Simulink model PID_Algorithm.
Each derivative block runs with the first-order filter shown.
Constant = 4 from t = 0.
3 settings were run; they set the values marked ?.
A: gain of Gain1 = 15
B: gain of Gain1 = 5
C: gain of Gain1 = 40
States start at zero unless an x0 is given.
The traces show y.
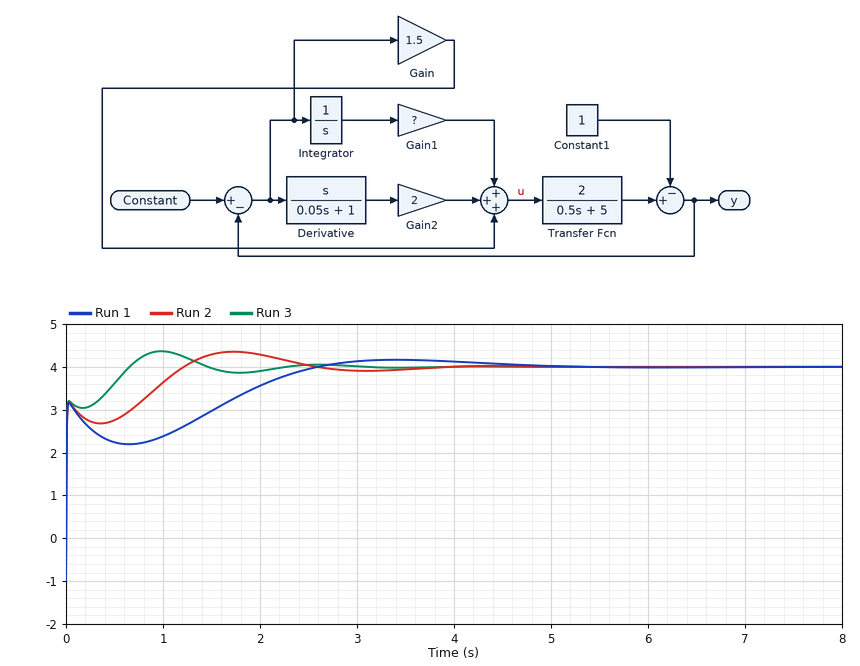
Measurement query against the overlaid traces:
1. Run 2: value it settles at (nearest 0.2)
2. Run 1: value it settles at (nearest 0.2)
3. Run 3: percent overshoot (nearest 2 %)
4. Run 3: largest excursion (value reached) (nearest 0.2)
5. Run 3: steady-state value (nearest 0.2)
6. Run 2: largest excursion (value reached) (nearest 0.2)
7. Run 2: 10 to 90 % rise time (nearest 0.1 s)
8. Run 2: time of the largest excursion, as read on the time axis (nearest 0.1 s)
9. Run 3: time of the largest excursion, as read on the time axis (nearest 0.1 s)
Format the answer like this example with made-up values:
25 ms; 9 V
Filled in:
4.0; 4.0; 8 %; 4.4; 4.0; 4.4; 0.9 s; 1.7 s; 1.0 s
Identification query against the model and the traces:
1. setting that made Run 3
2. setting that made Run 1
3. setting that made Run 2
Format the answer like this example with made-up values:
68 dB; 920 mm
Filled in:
C; B; A
